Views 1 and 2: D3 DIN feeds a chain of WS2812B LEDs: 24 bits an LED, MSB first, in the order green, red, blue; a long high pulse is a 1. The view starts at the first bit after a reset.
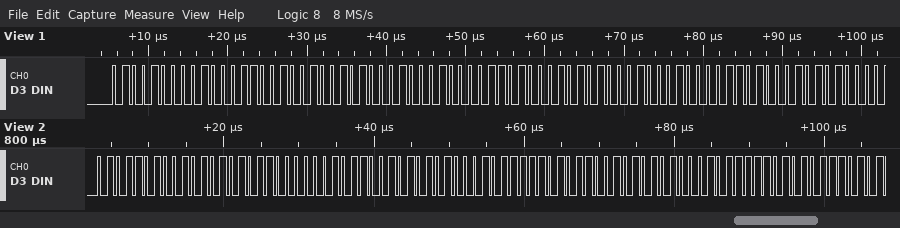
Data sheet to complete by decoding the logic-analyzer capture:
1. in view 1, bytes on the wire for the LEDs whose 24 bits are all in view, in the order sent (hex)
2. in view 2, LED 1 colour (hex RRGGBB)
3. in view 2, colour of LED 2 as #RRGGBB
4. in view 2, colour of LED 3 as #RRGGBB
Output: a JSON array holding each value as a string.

["48 46 49 44 43 45 44 43 45", "#555A60", "#54595F", "#54595F"]
